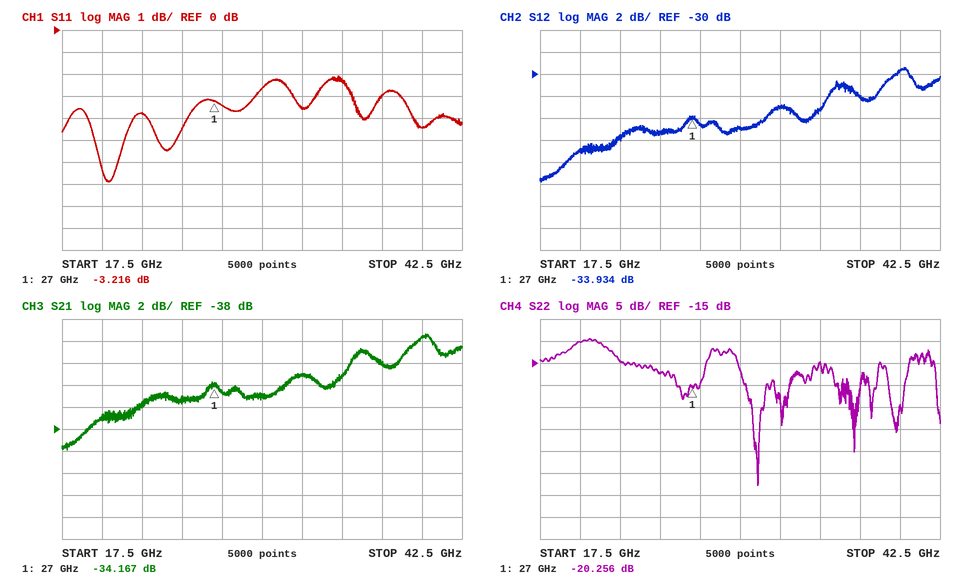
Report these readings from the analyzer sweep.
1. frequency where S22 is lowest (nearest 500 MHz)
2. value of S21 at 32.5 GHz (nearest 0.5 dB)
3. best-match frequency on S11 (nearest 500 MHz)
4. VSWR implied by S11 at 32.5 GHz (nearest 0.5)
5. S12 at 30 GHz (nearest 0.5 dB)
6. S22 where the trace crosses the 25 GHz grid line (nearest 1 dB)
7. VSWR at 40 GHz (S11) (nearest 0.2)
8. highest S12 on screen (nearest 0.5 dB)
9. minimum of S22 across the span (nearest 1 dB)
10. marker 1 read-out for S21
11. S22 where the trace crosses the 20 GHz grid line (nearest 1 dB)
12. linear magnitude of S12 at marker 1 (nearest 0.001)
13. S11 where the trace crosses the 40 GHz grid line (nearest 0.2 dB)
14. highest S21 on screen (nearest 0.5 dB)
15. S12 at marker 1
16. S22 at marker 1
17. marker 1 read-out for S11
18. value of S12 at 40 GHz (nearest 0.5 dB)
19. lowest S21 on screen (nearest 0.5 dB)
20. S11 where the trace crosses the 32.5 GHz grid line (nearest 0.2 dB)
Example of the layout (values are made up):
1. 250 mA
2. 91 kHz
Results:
1. 31.0 GHz
2. -33.0 dB
3. 20.5 GHz
4. 5.0
5. -35.0 dB
6. -17 dB
7. 4.0
8. -29.5 dB
9. -43 dB
10. -34.167 dB
11. -10 dB
12. 0.020
13. -4.4 dB
14. -29.5 dB
15. -33.934 dB
16. -20.256 dB
17. -3.216 dB
18. -29.5 dB
19. -40.0 dB
20. -3.6 dB
